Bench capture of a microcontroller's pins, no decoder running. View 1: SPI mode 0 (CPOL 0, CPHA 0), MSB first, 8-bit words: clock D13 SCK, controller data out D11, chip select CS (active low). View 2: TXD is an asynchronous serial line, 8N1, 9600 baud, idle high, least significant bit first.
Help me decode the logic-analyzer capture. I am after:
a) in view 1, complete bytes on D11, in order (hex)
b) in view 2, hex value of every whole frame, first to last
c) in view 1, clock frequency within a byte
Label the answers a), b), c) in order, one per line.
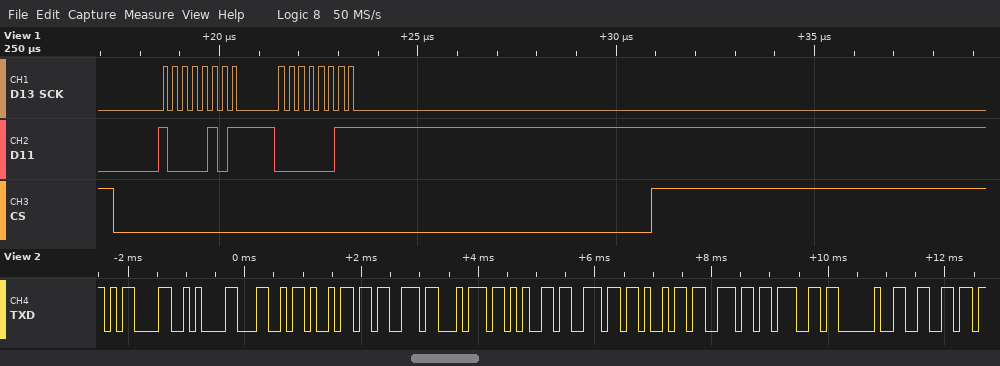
a) 85 03
b) 0D 0A 4C 69 73 74 65 6E 69 6E 67 20 66
c) 4 MHz
